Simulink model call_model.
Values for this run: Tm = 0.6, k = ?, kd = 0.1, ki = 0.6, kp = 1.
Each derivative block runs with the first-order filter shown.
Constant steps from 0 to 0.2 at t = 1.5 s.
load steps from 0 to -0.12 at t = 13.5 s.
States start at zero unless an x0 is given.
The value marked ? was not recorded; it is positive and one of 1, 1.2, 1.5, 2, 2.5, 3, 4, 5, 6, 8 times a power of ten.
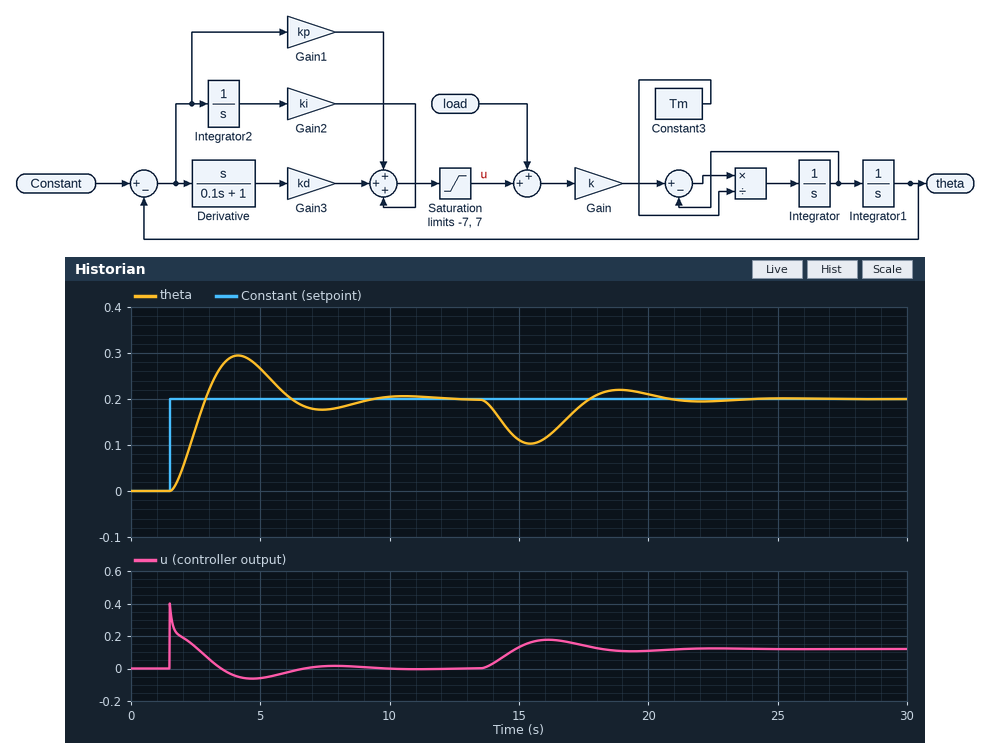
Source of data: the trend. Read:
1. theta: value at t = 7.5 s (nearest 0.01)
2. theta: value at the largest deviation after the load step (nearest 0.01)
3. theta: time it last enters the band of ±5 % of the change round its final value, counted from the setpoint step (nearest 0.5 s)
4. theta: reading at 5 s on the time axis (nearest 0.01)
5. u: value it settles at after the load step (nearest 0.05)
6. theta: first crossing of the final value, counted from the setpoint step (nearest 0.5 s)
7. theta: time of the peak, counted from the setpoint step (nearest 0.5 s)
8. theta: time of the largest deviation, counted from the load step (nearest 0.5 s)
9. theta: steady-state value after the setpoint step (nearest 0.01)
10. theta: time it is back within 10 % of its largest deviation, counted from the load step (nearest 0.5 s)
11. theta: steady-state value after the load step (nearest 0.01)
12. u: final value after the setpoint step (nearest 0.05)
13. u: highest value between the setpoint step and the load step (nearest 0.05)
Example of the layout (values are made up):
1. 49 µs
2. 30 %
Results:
1. 0.18
2. 0.10
3. 7.0 s
4. 0.27
5. 0.10
6. 1.5 s
7. 2.5 s
8. 2.0 s
9. 0.20
10. 6.5 s
11. 0.20
12. 0.00
13. 0.40
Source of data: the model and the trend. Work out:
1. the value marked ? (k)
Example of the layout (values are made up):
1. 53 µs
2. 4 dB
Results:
1. 1.2
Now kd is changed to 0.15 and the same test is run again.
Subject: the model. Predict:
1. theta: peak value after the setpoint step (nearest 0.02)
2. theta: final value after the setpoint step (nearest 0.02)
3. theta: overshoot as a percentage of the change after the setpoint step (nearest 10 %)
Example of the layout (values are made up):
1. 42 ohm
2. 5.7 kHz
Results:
1. 0.28
2. 0.20
3. 40 %
